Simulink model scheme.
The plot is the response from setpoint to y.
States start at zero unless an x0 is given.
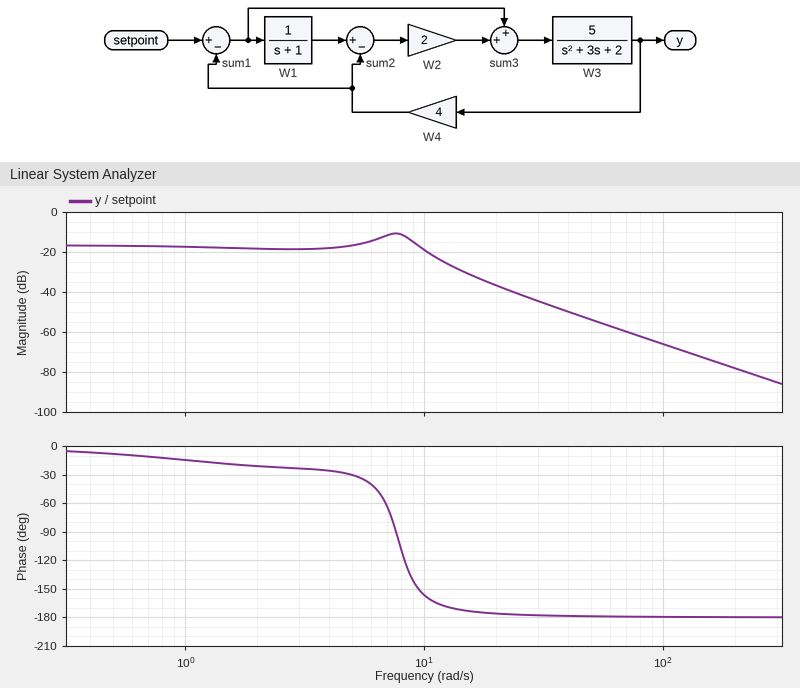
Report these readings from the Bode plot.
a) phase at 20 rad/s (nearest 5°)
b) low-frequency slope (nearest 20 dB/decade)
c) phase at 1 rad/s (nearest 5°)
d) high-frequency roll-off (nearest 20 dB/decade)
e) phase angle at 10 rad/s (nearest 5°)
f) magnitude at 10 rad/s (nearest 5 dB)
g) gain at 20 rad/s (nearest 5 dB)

-175°
0 dB/decade
-15°
-40 dB/decade
-155°
-20 dB
-35 dB
